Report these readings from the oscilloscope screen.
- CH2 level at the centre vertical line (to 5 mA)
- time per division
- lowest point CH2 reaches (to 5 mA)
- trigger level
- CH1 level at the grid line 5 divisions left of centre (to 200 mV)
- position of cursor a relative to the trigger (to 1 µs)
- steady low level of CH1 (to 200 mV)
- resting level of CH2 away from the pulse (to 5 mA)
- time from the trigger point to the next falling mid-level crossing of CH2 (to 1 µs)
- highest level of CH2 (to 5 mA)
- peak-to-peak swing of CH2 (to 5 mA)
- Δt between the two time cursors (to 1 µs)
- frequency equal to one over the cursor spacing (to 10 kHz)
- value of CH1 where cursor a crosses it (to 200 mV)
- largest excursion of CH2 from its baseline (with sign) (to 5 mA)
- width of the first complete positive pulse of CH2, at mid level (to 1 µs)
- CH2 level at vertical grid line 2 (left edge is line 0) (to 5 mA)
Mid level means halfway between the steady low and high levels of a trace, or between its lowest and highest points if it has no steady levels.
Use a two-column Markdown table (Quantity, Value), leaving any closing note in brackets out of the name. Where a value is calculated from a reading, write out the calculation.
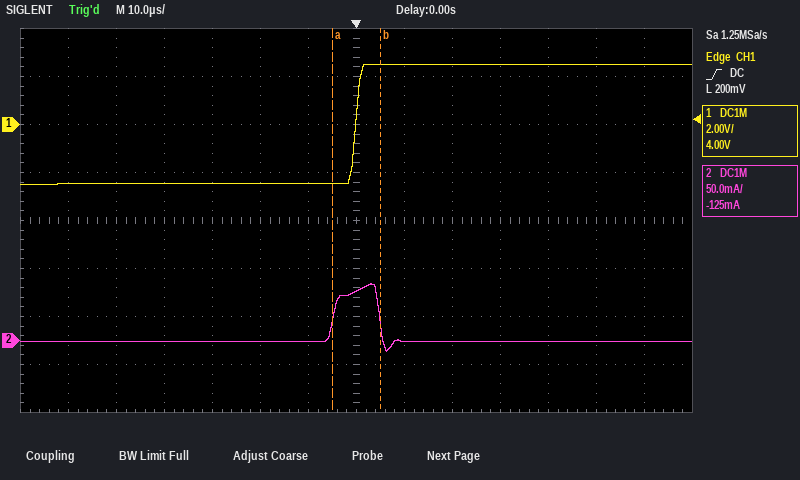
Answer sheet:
| Quantity | Value |
|---|---|
| CH2 level at the centre vertical line | 50 mA |
| time per division | 10 µs |
| lowest point CH2 reaches | -10 mA |
| trigger level | 200 mV |
| CH1 level at the grid line 5 divisions left of centre | -2.4 V |
| position of cursor a relative to the trigger | -5 µs |
| steady low level of CH1 | -2.4 V |
| resting level of CH2 away from the pulse | 0 mA |
| time from the trigger point to the next falling mid-level crossing of CH2 | 5 µs |
| highest level of CH2 | 60 mA |
| peak-to-peak swing of CH2 | 60 mA − (-10 mA) = 70 mA |
| Δt between the two time cursors | 10 µs |
| frequency equal to one over the cursor spacing | 1 / 10 µs ≈ 100 kHz |
| value of CH1 where cursor a crosses it | -2.4 V |
| largest excursion of CH2 from its baseline (with sign) | 60 mA − (0 mA) = +60 mA |
| width of the first complete positive pulse of CH2, at mid level | 10 µs |
| CH2 level at vertical grid line 2 (left edge is line 0) | 0 mA |
